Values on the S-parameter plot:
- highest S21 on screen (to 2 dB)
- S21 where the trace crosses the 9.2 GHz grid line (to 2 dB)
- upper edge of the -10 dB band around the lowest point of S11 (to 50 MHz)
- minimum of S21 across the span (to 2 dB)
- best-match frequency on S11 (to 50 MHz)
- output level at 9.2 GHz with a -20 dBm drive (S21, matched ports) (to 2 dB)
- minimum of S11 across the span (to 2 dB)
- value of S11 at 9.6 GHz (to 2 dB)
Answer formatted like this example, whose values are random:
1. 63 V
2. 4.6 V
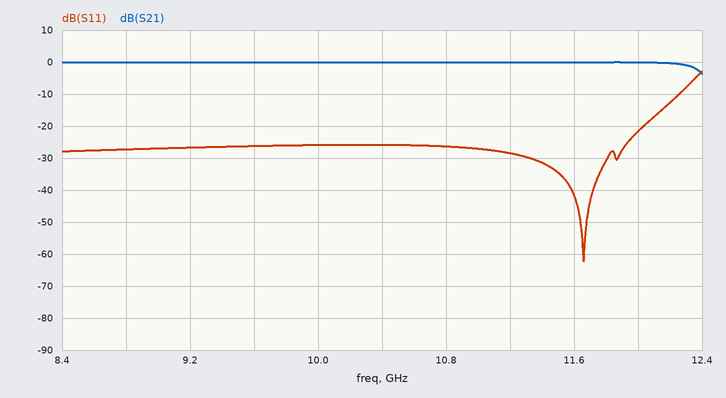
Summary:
1. 0 dB
2. 0 dB
3. 12.25 GHz
4. -4 dB
5. 11.65 GHz
6. -20 dBm
7. -62 dB
8. -26 dB
